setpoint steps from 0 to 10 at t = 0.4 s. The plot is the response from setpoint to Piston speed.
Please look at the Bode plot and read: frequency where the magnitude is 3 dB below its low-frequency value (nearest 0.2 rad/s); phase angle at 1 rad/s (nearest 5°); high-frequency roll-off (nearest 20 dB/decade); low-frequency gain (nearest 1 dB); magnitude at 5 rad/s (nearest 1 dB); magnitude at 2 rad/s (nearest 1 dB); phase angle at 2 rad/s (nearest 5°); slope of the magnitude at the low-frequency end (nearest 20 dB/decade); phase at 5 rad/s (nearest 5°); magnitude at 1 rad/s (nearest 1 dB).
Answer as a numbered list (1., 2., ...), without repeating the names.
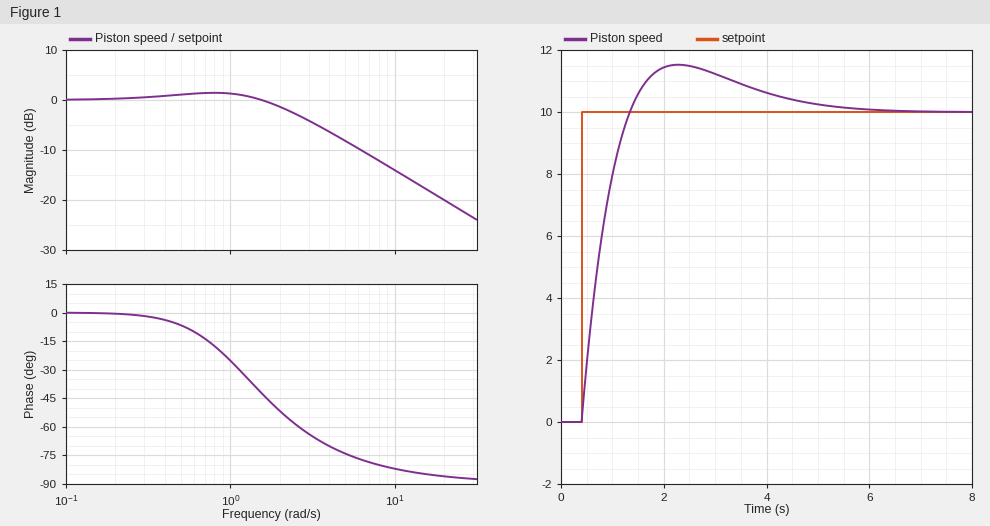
1. 2.6 rad/s
2. -25°
3. -20 dB/decade
4. 0 dB
5. -8 dB
6. -1 dB
7. -50°
8. 0 dB/decade
9. -75°
10. 1 dB
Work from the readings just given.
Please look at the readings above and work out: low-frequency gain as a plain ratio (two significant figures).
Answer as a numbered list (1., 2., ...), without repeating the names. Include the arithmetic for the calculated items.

1. 10^(0 / 20) = 1.0
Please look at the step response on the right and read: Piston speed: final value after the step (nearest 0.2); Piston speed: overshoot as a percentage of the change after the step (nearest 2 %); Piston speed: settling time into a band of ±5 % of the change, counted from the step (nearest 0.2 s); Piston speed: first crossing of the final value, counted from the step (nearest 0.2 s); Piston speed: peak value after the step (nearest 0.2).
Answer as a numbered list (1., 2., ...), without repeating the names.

1. 10.0
2. 16 %
3. 3.8 s
4. 1.0 s
5. 11.6
